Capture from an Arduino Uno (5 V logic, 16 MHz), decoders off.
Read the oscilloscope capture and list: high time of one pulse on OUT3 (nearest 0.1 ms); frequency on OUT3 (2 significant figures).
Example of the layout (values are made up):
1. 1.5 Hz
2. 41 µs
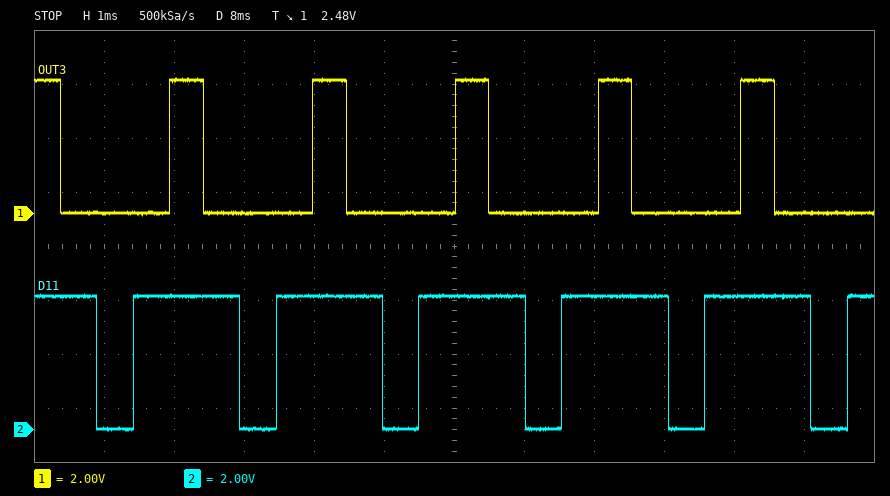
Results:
1. 0.5 ms
2. 490 Hz
